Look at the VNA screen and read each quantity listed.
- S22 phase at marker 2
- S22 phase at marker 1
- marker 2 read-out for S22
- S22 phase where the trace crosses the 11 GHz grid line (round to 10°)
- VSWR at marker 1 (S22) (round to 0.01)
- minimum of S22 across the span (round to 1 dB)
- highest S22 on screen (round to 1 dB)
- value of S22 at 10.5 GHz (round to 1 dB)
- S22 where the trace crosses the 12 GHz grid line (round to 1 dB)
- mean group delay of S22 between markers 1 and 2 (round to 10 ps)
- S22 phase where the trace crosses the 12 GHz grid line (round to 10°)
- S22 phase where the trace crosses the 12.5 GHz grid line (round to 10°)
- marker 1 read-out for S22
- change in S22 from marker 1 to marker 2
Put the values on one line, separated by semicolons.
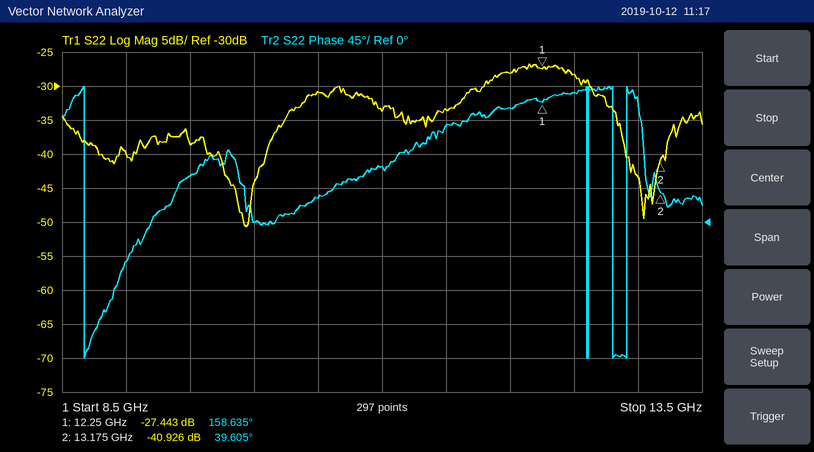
39.605°; 158.635°; -40.926 dB; 70°; 1.09; -51 dB; -27 dB; -31 dB; -28 dB; 360 ps; 150°; 170°; -27.443 dB; -13.483 dB
